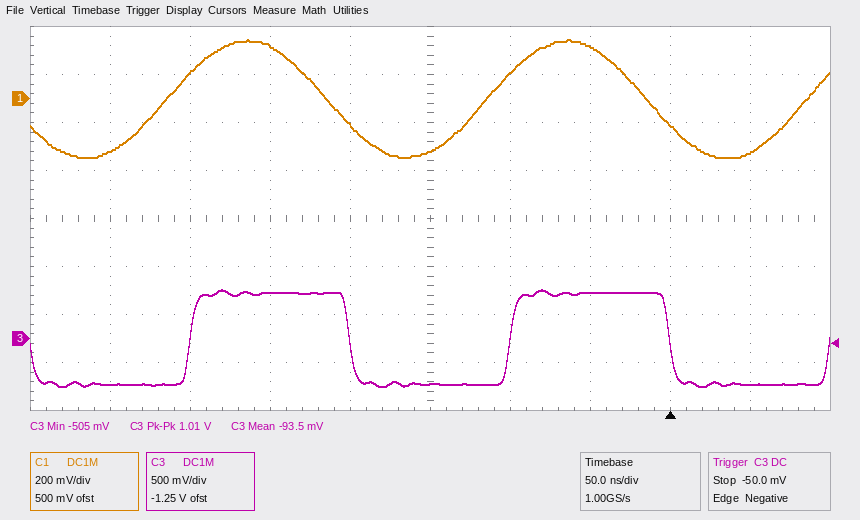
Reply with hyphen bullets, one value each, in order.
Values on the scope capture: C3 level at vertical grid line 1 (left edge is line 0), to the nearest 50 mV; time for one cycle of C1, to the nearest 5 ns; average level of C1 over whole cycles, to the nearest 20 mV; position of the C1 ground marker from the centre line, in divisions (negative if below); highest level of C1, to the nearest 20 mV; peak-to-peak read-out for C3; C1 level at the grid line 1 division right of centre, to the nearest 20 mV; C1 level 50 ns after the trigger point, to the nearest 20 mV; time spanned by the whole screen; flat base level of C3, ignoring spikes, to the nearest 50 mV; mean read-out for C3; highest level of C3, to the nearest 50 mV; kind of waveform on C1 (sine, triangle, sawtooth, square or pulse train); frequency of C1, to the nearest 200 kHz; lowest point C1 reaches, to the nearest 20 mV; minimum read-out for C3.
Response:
- -500 mV
- 200 ns
- 0 mV
- +2.5 div
- 240 mV
- 1.01 V
- 100 mV
- -220 mV
- 500 ns
- -500 mV
- -93.5 mV
- 500 mV
- sine
- 5.0 MHz
- -240 mV
- -505 mV
